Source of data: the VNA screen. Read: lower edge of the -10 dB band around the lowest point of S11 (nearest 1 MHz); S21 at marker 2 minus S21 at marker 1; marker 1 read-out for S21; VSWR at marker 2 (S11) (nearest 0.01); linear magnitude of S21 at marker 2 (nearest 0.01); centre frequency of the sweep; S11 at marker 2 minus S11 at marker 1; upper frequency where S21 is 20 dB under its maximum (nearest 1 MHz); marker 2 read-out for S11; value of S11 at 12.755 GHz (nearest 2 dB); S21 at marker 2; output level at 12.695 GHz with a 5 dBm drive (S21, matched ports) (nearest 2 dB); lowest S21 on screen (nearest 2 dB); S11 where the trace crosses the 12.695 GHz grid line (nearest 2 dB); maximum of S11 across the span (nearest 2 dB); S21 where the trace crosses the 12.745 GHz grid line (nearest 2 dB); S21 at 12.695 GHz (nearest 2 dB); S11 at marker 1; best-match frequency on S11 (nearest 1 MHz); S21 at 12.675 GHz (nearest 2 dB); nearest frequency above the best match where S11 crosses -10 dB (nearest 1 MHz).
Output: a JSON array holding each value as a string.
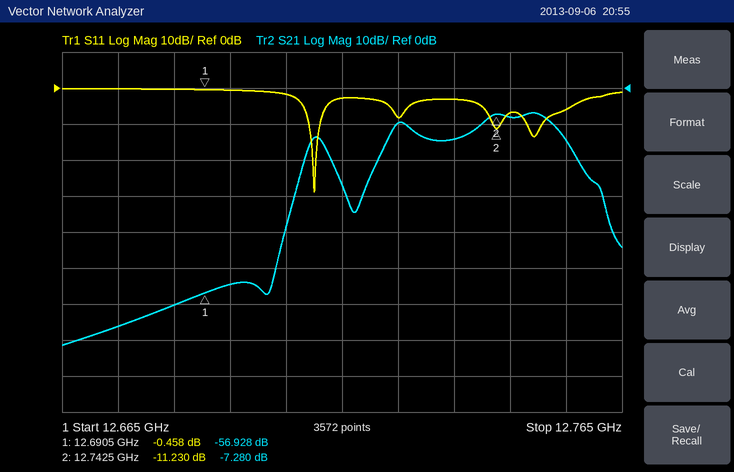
["12.709 GHz", "49.648 dB", "-56.928 dB", "1.76", "0.43", "12.715 GHz", "-10.772 dB", "12.761 GHz", "-11.230 dB", "-6 dB", "-7.280 dB", "-50 dBm", "-72 dB", "0 dB", "0 dB", "-8 dB", "-54 dB", "-0.458 dB", "12.710 GHz", "-66 dB", "12.711 GHz"]
